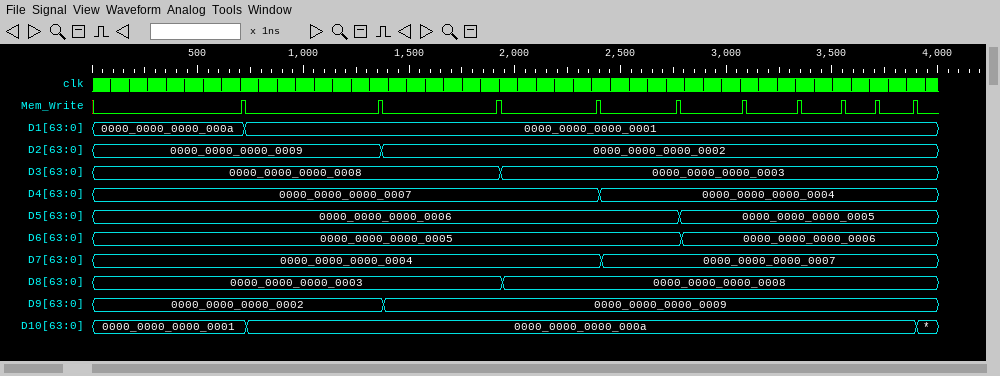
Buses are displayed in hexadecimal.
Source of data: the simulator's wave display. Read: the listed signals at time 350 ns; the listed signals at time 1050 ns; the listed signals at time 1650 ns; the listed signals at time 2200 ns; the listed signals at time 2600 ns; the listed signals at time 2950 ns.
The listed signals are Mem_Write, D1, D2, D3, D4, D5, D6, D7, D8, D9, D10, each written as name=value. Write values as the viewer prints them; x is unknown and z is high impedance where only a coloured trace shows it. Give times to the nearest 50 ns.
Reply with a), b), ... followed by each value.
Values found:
a) Mem_Write=0, D1=0000_0000_0000_000a, D2=0000_0000_0000_0009, D3=0000_0000_0000_0008, D4=0000_0000_0000_0007, D5=0000_0000_0000_0006, D6=0000_0000_0000_0005, D7=0000_0000_0000_0004, D8=0000_0000_0000_0003, D9=0000_0000_0000_0002, D10=0000_0000_0000_0001
b) Mem_Write=0, D1=0000_0000_0000_0001, D2=0000_0000_0000_0009, D3=0000_0000_0000_0008, D4=0000_0000_0000_0007, D5=0000_0000_0000_0006, D6=0000_0000_0000_0005, D7=0000_0000_0000_0004, D8=0000_0000_0000_0003, D9=0000_0000_0000_0002, D10=0000_0000_0000_000a
c) Mem_Write=0, D1=0000_0000_0000_0001, D2=0000_0000_0000_0002, D3=0000_0000_0000_0008, D4=0000_0000_0000_0007, D5=0000_0000_0000_0006, D6=0000_0000_0000_0005, D7=0000_0000_0000_0004, D8=0000_0000_0000_0003, D9=0000_0000_0000_0009, D10=0000_0000_0000_000a
d) Mem_Write=0, D1=0000_0000_0000_0001, D2=0000_0000_0000_0002, D3=0000_0000_0000_0003, D4=0000_0000_0000_0007, D5=0000_0000_0000_0006, D6=0000_0000_0000_0005, D7=0000_0000_0000_0004, D8=0000_0000_0000_0008, D9=0000_0000_0000_0009, D10=0000_0000_0000_000a
e) Mem_Write=0, D1=0000_0000_0000_0001, D2=0000_0000_0000_0002, D3=0000_0000_0000_0003, D4=0000_0000_0000_0004, D5=0000_0000_0000_0006, D6=0000_0000_0000_0005, D7=0000_0000_0000_0007, D8=0000_0000_0000_0008, D9=0000_0000_0000_0009, D10=0000_0000_0000_000a
f) Mem_Write=0, D1=0000_0000_0000_0001, D2=0000_0000_0000_0002, D3=0000_0000_0000_0003, D4=0000_0000_0000_0004, D5=0000_0000_0000_0005, D6=0000_0000_0000_0006, D7=0000_0000_0000_0007, D8=0000_0000_0000_0008, D9=0000_0000_0000_0009, D10=0000_0000_0000_000a
